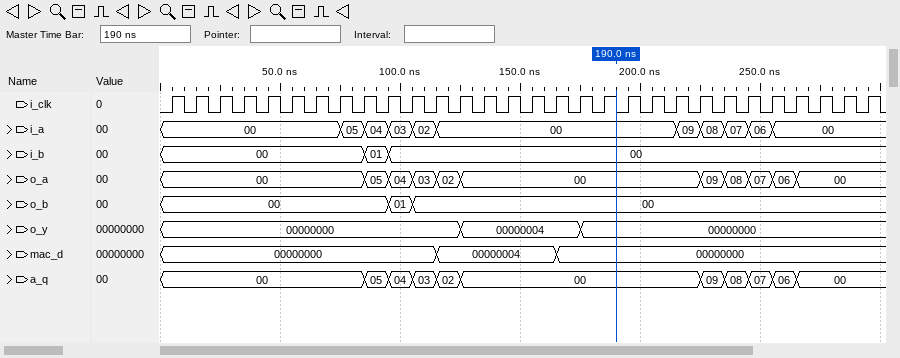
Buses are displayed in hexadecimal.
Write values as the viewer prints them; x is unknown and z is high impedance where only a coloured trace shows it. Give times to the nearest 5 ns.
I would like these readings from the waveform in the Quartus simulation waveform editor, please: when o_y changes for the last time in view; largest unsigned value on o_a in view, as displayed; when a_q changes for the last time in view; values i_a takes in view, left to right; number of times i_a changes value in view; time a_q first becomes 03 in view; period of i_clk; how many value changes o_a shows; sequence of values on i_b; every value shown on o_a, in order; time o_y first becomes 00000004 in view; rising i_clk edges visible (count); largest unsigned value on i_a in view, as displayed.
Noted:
175 ns
09
265 ns
00, 05, 04, 03, 02, 00, 09, 08, 07, 06, 00
10
105 ns
10 ns
10
00, 01, 00
00, 05, 04, 03, 02, 00, 09, 08, 07, 06, 00
125 ns
30
09
